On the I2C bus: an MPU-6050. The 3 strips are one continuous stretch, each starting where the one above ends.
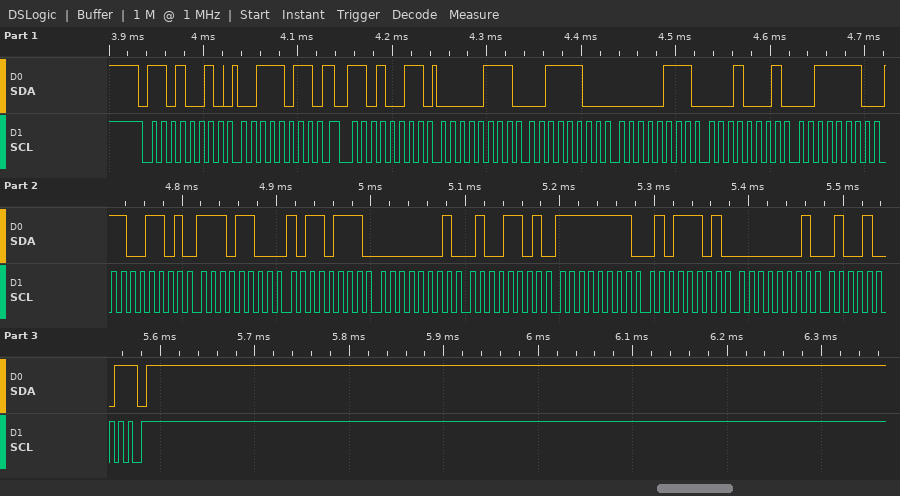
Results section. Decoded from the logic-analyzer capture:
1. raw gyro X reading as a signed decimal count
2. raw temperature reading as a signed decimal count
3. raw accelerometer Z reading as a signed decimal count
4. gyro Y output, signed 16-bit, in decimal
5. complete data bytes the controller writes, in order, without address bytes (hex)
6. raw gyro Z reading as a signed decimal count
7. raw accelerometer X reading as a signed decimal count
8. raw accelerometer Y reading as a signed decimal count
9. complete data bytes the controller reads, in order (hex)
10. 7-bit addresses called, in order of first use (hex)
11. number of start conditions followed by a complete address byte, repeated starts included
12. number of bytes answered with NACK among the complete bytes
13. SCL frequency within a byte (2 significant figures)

333
-4937
16077
-163
3B
329
1852
1809
07 3C 07 11 3E CD EC B7 01 4D FF 5D 01 49
0x69
2
1
100 kHz
